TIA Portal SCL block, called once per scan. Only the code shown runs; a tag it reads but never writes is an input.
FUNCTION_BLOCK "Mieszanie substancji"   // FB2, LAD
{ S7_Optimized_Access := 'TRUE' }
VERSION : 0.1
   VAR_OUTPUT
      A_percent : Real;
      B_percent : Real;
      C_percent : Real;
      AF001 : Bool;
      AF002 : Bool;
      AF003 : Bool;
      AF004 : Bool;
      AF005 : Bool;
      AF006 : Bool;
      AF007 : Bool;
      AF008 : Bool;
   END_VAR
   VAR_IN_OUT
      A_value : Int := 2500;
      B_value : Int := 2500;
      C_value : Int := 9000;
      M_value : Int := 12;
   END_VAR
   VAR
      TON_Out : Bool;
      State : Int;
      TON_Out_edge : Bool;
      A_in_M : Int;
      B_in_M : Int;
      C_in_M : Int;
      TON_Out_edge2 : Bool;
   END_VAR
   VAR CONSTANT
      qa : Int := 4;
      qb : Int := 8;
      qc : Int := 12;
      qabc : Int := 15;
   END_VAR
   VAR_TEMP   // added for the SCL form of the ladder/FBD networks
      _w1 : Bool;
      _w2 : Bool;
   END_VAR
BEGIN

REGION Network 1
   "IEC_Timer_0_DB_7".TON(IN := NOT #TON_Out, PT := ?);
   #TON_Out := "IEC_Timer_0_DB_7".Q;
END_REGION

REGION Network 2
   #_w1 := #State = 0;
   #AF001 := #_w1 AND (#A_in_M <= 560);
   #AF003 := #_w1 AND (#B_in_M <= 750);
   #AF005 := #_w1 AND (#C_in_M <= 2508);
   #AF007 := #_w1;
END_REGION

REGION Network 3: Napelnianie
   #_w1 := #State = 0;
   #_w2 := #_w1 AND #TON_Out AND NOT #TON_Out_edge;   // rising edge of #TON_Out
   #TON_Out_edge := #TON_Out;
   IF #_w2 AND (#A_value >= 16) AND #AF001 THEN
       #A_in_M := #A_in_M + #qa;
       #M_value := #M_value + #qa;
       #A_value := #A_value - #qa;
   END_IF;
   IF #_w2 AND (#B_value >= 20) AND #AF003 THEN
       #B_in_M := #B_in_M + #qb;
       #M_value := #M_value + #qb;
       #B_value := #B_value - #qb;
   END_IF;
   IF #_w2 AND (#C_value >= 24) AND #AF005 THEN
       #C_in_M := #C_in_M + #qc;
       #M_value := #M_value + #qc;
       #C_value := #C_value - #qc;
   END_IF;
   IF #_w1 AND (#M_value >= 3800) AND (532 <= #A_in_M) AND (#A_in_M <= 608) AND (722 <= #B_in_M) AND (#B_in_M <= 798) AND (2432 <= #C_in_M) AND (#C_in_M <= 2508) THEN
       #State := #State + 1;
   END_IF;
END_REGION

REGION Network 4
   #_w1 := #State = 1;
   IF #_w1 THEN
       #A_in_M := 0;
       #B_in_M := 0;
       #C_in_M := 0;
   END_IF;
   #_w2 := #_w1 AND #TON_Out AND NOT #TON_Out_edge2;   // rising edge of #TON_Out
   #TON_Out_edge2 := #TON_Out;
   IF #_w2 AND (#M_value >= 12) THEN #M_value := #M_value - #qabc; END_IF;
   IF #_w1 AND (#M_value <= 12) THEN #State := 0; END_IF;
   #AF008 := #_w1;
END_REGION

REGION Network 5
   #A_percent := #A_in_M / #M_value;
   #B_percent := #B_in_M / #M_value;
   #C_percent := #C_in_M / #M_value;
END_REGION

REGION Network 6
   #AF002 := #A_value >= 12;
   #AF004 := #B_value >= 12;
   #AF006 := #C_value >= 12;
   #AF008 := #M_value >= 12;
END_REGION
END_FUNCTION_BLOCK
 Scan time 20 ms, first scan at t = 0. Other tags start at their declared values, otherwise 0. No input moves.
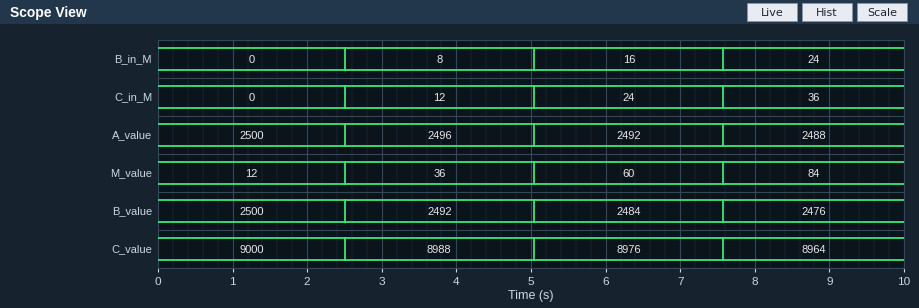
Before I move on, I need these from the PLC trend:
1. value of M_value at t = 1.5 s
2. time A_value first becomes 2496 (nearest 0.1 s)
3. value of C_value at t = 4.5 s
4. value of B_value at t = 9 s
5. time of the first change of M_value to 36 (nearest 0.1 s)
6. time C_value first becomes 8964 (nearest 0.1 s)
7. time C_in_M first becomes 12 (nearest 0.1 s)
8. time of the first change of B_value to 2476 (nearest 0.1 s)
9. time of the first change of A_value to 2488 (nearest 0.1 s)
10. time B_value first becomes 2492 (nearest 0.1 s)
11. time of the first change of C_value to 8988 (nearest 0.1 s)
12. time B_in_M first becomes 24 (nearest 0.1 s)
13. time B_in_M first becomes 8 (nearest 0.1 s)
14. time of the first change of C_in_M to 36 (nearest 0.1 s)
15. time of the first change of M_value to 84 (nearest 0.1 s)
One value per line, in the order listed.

12
2.5 s
8988
2476
2.5 s
7.6 s
2.5 s
7.6 s
7.6 s
2.5 s
2.5 s
7.6 s
2.5 s
7.6 s
7.6 s
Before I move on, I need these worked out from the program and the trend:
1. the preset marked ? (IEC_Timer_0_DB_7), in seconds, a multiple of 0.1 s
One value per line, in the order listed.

2.5 s
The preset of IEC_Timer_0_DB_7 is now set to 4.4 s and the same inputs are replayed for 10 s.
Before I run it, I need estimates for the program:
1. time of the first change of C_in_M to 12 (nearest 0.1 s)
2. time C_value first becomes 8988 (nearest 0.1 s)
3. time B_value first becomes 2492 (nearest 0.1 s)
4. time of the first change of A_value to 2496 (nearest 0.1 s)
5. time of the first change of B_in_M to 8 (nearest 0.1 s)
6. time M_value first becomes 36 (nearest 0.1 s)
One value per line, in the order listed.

4.4 s
4.4 s
4.4 s
4.4 s
4.4 s
4.4 s
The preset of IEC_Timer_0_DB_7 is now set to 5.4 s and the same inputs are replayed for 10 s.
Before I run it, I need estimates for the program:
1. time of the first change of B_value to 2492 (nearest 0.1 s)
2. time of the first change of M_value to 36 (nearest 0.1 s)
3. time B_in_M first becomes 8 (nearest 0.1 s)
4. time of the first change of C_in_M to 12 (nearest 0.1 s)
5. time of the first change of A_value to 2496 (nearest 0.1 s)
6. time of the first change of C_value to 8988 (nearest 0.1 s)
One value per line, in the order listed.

5.4 s
5.4 s
5.4 s
5.4 s
5.4 s
5.4 s
